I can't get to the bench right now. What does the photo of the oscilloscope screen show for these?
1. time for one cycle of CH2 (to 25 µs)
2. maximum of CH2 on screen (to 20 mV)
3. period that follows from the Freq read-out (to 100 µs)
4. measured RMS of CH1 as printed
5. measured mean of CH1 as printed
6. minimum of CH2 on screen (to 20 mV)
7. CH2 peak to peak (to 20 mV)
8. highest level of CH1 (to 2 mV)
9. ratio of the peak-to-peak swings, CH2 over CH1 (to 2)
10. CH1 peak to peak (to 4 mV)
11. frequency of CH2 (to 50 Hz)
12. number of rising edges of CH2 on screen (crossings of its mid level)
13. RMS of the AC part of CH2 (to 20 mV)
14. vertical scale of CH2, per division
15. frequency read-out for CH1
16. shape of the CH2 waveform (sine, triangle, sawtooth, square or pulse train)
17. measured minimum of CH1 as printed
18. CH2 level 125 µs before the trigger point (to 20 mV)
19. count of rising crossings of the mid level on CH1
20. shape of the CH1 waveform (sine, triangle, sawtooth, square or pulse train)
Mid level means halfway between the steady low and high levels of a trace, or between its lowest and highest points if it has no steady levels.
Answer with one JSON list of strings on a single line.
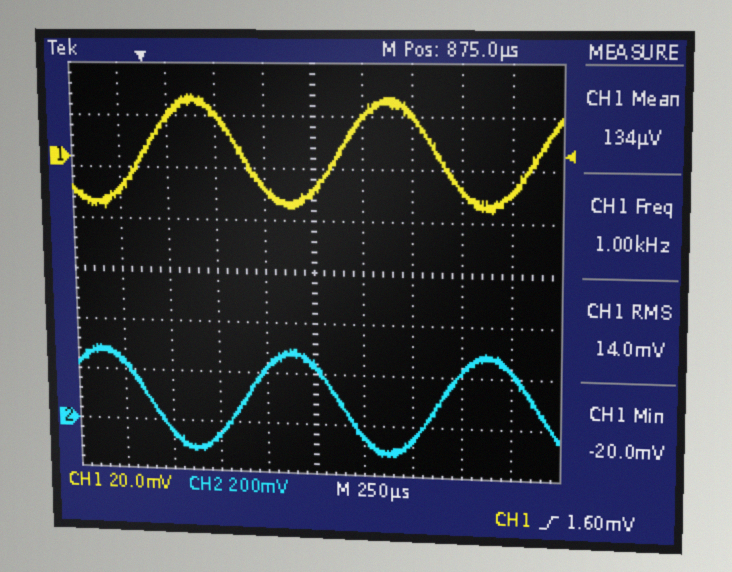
["1.000 ms", "300 mV", "1.0 ms", "14.0 mV", "134 µV", "-120 mV", "420 mV", "24 mV", "10", "44 mV", "1.00 kHz", "2", "140 mV", "200 mV", "1.00 kHz", "sine", "-20.0 mV", "220 mV", "3", "sine"]
